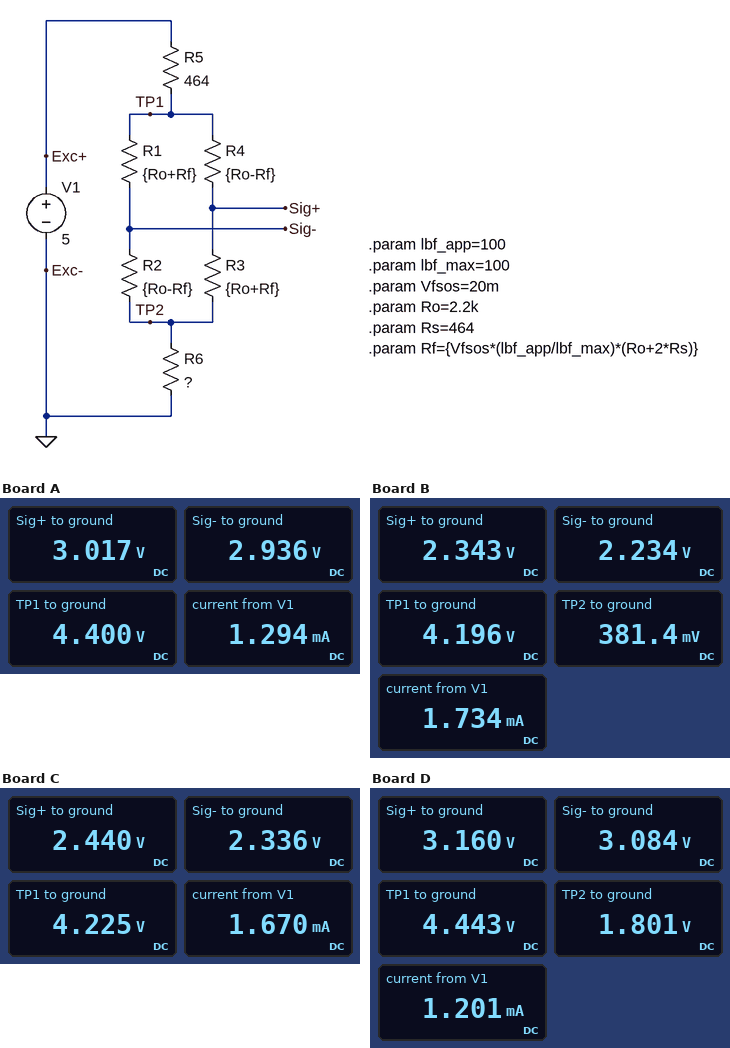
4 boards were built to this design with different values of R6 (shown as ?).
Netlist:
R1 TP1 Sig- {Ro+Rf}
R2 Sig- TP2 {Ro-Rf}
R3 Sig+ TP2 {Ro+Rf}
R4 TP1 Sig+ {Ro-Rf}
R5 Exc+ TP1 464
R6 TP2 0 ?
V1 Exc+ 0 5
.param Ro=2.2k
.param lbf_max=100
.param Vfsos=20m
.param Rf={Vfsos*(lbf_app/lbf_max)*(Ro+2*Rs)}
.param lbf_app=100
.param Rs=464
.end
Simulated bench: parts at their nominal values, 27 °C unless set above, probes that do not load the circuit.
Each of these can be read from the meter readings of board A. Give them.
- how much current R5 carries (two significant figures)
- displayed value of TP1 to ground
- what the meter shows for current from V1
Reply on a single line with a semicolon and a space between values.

1.3 mA; 4.400 V; 1.294 mA
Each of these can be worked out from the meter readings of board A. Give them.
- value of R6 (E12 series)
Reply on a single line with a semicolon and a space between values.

1.2 kΩ
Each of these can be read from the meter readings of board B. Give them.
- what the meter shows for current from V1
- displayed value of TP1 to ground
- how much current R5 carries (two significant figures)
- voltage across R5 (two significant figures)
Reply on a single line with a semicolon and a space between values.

1.734 mA; 4.196 V; 1.7 mA; 800 mV
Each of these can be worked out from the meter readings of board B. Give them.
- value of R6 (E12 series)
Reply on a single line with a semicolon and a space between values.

220 Ω
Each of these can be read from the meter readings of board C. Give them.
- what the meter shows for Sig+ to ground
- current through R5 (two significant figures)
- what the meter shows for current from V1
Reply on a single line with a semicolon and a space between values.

2.440 V; 1.7 mA; 1.670 mA
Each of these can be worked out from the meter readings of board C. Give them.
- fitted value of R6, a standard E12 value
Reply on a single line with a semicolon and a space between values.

330 Ω
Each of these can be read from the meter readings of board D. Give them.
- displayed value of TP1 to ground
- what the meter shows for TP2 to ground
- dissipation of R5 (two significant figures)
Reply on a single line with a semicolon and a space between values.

4.443 V; 1.801 V; 670 µW
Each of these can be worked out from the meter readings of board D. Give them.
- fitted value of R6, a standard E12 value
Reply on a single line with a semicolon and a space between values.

1.5 kΩ
